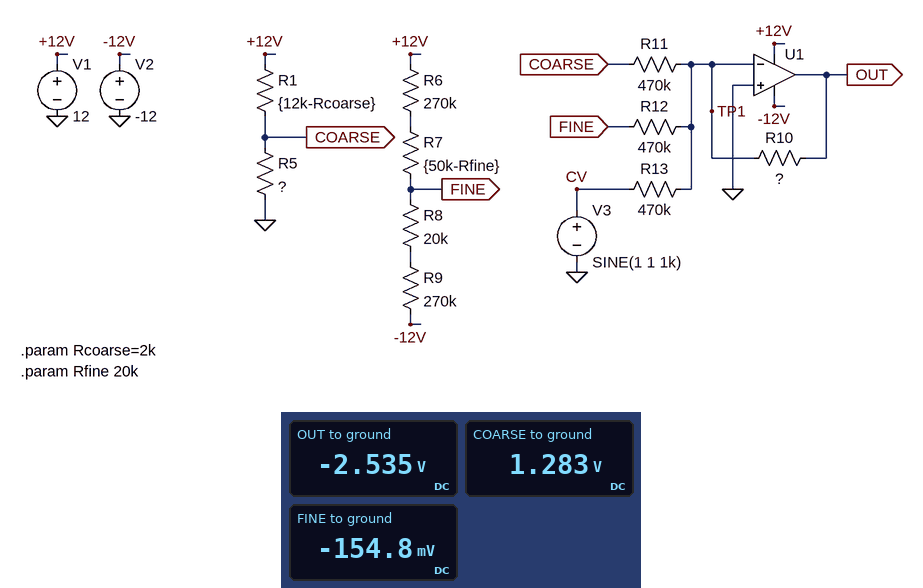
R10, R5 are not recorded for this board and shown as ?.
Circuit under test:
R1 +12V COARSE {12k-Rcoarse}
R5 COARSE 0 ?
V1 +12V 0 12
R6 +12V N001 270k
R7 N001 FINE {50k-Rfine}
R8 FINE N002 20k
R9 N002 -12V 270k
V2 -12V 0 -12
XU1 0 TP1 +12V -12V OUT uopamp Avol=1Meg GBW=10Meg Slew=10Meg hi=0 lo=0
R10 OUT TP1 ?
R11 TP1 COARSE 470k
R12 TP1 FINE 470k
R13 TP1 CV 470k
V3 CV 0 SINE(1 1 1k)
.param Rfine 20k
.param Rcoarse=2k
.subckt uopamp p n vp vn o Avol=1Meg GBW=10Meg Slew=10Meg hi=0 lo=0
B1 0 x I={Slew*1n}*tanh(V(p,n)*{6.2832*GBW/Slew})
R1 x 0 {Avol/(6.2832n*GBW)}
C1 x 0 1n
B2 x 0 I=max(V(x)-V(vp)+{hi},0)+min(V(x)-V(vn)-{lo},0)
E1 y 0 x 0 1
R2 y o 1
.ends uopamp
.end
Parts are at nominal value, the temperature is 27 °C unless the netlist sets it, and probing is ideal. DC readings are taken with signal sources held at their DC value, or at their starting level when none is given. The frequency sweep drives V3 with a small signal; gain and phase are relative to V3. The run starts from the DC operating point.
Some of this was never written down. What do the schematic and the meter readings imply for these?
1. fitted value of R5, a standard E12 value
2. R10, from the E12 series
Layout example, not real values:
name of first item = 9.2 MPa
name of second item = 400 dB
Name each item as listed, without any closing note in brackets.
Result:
fitted value of R5, a standard E12 value = 1.2 kΩ
R10, from the E12 series = 560 kΩ
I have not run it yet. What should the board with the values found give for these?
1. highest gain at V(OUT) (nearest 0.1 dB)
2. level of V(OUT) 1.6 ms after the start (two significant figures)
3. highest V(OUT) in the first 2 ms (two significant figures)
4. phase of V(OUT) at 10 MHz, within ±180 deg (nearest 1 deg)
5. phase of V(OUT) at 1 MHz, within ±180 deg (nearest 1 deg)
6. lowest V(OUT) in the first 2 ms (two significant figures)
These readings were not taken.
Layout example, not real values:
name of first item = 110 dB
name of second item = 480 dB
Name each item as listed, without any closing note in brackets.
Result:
highest gain at V(OUT) = 1.5 dB
level of V(OUT) 1.6 ms after the start = -1.8 V
highest V(OUT) in the first 2 ms = -1.3 V
phase of V(OUT) at 10 MHz, within ±180 deg = 103 deg
phase of V(OUT) at 1 MHz, within ±180 deg = 157 deg
lowest V(OUT) in the first 2 ms = -3.7 V
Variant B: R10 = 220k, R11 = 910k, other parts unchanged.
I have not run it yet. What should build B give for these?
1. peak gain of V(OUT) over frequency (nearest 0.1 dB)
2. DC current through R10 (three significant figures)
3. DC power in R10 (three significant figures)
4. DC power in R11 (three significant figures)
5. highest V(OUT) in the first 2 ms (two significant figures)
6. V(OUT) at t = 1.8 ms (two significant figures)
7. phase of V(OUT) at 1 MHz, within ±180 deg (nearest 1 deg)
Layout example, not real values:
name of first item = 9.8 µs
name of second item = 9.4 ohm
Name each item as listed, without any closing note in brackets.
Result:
peak gain of V(OUT) over frequency = -6.6 dB
DC current through R10 = 3.21 µA
DC power in R10 = 2.27 µW
DC power in R11 = 1.81 µW
highest V(OUT) in the first 2 ms = -240 mV
V(OUT) at t = 1.8 ms = -260 mV
phase of V(OUT) at 1 MHz, within ±180 deg = 168 deg
